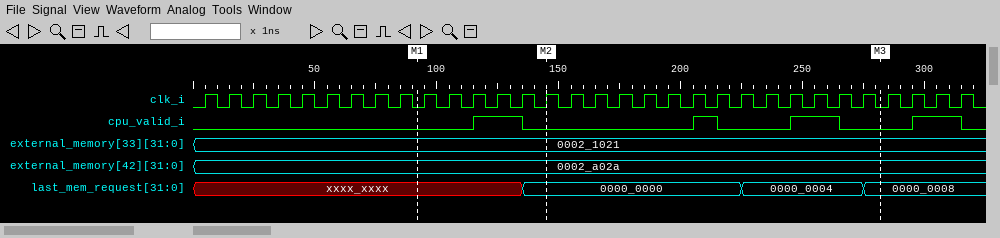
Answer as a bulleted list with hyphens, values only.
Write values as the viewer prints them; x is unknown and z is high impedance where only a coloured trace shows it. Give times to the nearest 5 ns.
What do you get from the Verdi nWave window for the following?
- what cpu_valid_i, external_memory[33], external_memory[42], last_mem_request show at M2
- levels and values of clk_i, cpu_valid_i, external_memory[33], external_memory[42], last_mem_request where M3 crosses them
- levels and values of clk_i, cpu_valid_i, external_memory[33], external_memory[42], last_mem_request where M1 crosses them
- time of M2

- cpu_valid_i=0, external_memory[33]=0002_1021, external_memory[42]=0002_a02a, last_mem_request=0000_0000
- clk_i=0, cpu_valid_i=0, external_memory[33]=0002_1021, external_memory[42]=0002_a02a, last_mem_request=0000_0008
- clk_i=0, cpu_valid_i=0, external_memory[33]=0002_1021, external_memory[42]=0002_a02a, last_mem_request=xxxx_xxxx
- 145 ns
